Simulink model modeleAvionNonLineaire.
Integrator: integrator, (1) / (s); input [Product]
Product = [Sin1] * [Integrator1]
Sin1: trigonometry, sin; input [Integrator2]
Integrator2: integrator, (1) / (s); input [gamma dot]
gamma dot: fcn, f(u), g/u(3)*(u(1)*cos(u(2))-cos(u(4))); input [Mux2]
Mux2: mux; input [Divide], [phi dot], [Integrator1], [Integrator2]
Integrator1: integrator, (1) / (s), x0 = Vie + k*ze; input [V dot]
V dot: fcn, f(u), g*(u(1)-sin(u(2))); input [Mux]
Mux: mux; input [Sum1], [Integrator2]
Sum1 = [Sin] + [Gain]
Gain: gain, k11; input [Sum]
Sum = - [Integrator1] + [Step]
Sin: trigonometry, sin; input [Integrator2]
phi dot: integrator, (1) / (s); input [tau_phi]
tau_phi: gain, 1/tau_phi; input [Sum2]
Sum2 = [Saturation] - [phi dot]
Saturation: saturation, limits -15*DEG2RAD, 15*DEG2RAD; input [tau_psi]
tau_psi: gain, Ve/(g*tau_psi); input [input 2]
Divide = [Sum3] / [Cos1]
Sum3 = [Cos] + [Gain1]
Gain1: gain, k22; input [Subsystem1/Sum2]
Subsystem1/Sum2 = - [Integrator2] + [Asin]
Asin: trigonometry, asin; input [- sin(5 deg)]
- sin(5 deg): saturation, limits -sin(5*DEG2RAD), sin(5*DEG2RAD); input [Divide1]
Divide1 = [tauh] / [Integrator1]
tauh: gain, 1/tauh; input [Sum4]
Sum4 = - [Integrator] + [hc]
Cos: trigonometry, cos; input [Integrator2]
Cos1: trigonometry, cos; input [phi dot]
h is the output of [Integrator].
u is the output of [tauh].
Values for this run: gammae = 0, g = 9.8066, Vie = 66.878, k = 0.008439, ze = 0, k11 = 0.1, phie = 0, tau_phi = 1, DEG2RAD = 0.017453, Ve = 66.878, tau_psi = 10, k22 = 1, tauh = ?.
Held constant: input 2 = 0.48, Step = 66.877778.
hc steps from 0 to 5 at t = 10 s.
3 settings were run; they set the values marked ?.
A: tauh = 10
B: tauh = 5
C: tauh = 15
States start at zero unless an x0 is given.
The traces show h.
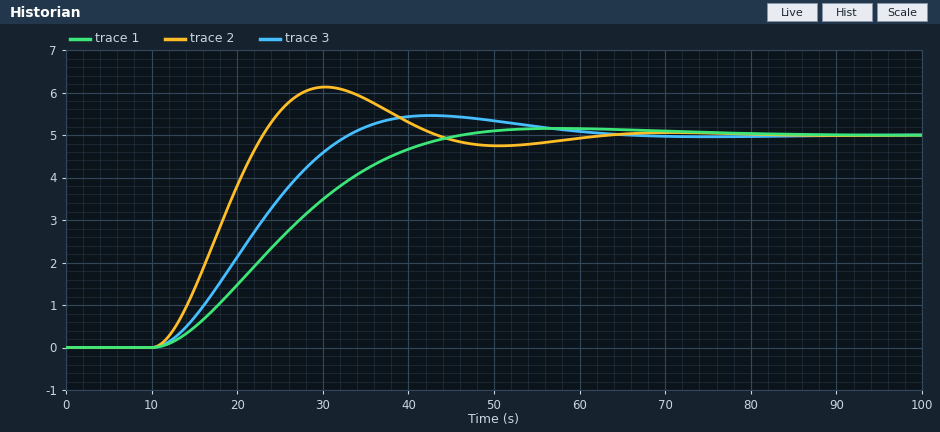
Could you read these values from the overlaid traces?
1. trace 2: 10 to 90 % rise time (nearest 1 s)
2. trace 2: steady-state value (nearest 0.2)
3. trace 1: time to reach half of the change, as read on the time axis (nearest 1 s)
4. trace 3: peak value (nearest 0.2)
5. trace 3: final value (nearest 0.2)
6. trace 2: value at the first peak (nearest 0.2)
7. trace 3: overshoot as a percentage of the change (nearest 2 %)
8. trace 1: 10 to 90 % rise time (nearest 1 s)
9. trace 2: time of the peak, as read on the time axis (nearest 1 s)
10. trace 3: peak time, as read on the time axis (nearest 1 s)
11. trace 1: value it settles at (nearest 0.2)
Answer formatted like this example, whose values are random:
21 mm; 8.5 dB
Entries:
9 s; 5.0; 25 s; 5.4; 5.0; 6.2; 10 %; 23 s; 30 s; 43 s; 5.0
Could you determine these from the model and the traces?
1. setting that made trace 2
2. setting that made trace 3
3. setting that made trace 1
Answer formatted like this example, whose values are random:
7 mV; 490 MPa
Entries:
B; A; C
